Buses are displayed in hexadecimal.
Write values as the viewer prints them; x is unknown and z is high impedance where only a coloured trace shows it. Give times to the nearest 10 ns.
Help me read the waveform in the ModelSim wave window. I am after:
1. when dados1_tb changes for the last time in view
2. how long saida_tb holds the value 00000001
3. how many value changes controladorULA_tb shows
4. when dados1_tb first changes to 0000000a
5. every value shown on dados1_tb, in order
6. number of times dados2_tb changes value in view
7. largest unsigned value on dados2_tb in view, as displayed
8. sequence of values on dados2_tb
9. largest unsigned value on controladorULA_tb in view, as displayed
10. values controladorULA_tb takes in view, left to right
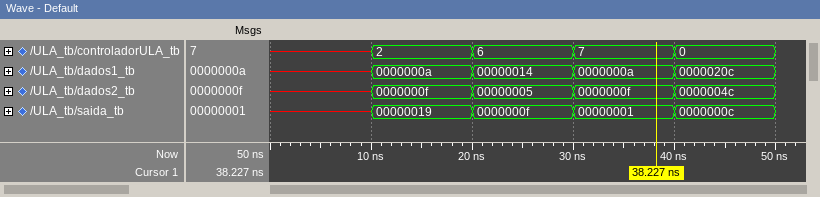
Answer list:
40 ns
10 ns
4
10 ns
x, 0000000a, 00000014, 0000000a, 0000020c
4
0000004c
x, 0000000f, 00000005, 0000000f, 0000004c
7
x, 2, 6, 7, 0
